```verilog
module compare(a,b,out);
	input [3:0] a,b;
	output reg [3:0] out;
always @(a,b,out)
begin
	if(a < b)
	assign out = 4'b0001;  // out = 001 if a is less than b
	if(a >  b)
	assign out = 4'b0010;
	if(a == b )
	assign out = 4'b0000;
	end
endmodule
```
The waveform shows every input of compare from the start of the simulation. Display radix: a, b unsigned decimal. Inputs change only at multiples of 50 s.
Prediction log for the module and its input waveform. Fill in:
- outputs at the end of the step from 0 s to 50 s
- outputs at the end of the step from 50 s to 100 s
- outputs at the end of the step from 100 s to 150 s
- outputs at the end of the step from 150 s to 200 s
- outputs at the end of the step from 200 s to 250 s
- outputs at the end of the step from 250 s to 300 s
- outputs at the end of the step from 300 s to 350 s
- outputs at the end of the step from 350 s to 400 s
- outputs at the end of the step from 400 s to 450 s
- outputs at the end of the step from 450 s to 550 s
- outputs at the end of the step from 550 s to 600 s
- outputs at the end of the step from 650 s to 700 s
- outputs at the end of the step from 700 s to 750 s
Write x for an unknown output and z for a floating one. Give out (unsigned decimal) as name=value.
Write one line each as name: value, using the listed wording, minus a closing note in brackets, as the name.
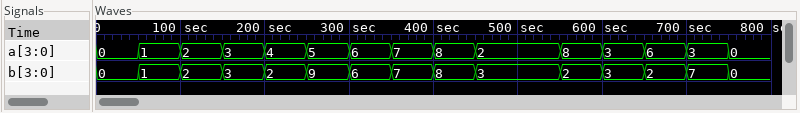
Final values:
outputs at the end of the step from 0 s to 50 s: out=0
outputs at the end of the step from 50 s to 100 s: out=0
outputs at the end of the step from 100 s to 150 s: out=0
outputs at the end of the step from 150 s to 200 s: out=0
outputs at the end of the step from 200 s to 250 s: out=2
outputs at the end of the step from 250 s to 300 s: out=1
outputs at the end of the step from 300 s to 350 s: out=0
outputs at the end of the step from 350 s to 400 s: out=0
outputs at the end of the step from 400 s to 450 s: out=0
outputs at the end of the step from 450 s to 550 s: out=1
outputs at the end of the step from 550 s to 600 s: out=2
outputs at the end of the step from 650 s to 700 s: out=2
outputs at the end of the step from 700 s to 750 s: out=1
